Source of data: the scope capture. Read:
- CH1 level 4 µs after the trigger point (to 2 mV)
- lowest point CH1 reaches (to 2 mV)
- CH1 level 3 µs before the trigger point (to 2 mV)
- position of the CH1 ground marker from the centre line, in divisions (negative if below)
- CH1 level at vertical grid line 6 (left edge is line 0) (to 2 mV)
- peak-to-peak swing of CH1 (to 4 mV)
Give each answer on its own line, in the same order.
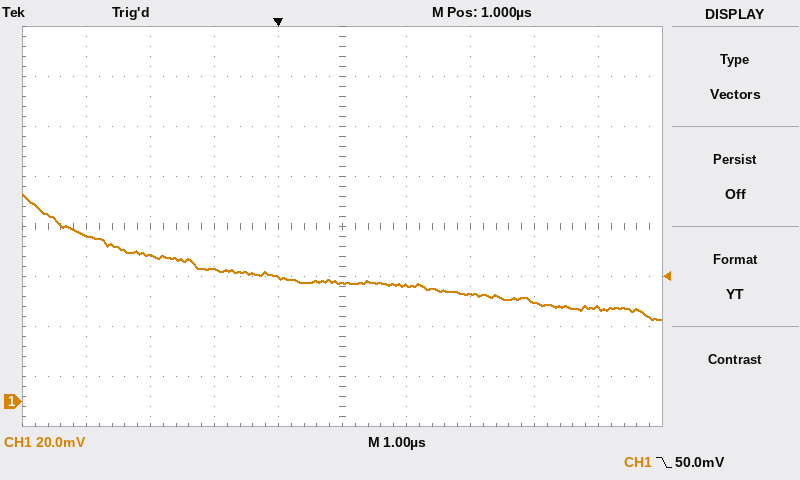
40 mV
32 mV
66 mV
-3.5 div
46 mV
52 mV
